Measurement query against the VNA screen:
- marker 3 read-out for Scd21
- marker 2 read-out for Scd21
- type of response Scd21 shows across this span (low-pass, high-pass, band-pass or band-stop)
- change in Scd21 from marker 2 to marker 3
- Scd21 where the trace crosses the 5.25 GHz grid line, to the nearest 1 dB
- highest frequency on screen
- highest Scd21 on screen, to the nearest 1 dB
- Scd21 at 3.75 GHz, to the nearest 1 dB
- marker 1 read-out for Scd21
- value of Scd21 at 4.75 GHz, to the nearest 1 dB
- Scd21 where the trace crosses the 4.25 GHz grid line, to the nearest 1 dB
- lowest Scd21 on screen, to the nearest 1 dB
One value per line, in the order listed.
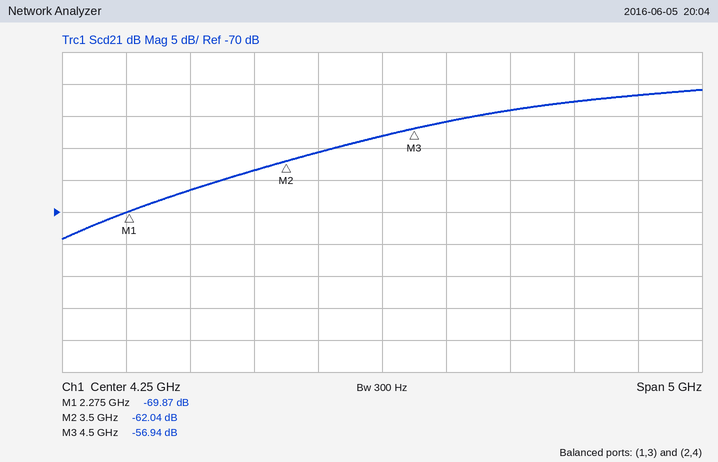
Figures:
-56.94 dB
-62.04 dB
high-pass
5.10 dB
-54 dB
6.75 GHz
-51 dB
-61 dB
-69.87 dB
-56 dB
-58 dB
-74 dB
